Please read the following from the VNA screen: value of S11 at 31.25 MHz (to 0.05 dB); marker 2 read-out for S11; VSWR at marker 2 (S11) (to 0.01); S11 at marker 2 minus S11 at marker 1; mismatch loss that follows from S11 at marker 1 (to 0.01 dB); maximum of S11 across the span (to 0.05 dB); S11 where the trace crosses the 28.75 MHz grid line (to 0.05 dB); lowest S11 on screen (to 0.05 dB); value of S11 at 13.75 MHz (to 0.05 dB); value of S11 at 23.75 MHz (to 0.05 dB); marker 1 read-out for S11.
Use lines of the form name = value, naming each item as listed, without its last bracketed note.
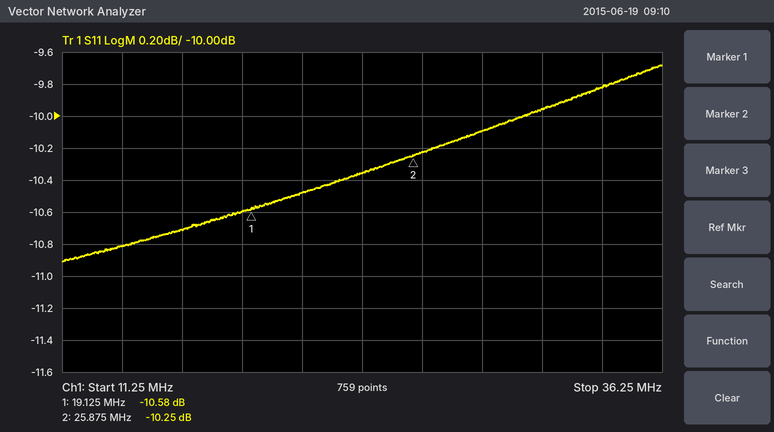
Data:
value of S11 at 31.25 MHz = -9.95 dB
marker 2 read-out for S11 = -10.25 dB
VSWR at marker 2 (S11) = 1.89
S11 at marker 2 minus S11 at marker 1 = 0.33 dB
mismatch loss that follows from S11 at marker 1 = 0.40 dB
maximum of S11 across the span = -9.70 dB
S11 where the trace crosses the 28.75 MHz grid line = -10.10 dB
lowest S11 on screen = -10.90 dB
value of S11 at 13.75 MHz = -10.80 dB
value of S11 at 23.75 MHz = -10.35 dB
marker 1 read-out for S11 = -10.58 dB
